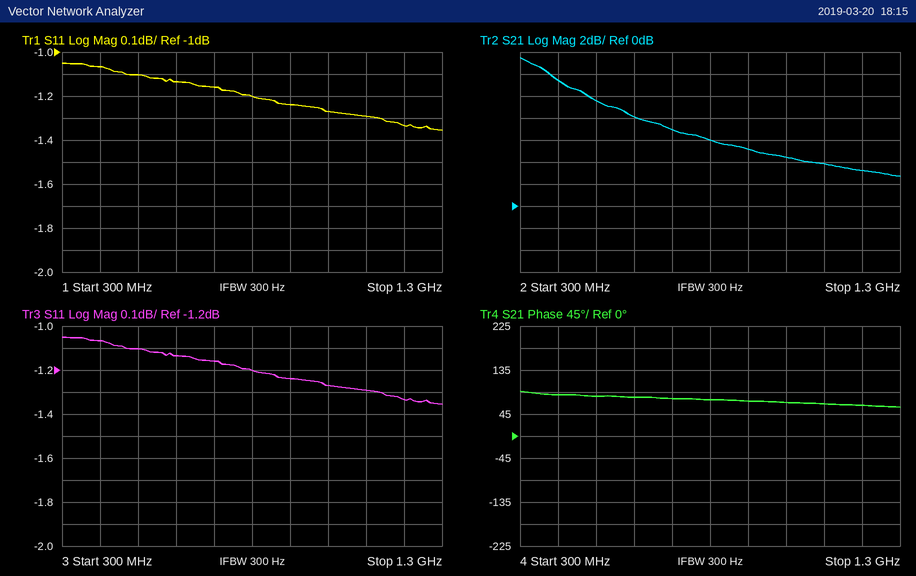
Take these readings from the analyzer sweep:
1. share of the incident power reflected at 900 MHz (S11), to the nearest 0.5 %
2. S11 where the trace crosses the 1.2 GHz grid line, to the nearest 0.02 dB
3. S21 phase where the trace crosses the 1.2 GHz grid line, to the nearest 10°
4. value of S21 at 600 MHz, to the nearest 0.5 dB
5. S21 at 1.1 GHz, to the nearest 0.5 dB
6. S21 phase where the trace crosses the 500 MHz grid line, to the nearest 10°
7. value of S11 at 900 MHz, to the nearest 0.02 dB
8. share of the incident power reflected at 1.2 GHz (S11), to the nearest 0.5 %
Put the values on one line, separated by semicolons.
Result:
75.0 %; -1.34 dB; 60°; 8.0 dB; 4.0 dB; 80°; -1.24 dB; 73.5 %
